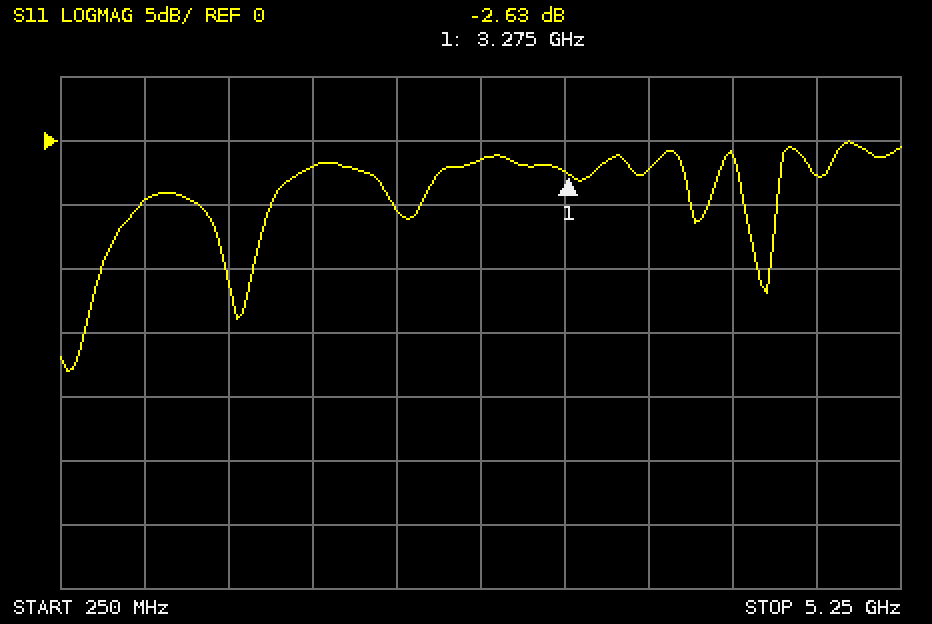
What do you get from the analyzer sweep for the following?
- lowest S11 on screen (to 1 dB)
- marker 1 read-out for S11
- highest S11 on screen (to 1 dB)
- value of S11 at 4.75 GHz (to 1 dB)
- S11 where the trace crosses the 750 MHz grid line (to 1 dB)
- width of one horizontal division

-18 dB
-2.63 dB
0 dB
-3 dB
-5 dB
500 MHz
